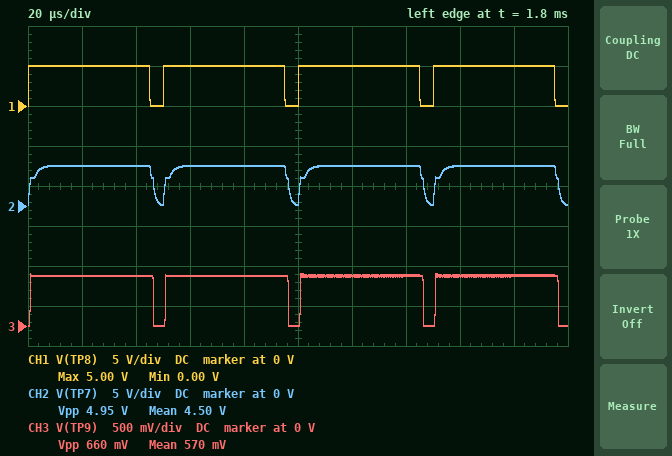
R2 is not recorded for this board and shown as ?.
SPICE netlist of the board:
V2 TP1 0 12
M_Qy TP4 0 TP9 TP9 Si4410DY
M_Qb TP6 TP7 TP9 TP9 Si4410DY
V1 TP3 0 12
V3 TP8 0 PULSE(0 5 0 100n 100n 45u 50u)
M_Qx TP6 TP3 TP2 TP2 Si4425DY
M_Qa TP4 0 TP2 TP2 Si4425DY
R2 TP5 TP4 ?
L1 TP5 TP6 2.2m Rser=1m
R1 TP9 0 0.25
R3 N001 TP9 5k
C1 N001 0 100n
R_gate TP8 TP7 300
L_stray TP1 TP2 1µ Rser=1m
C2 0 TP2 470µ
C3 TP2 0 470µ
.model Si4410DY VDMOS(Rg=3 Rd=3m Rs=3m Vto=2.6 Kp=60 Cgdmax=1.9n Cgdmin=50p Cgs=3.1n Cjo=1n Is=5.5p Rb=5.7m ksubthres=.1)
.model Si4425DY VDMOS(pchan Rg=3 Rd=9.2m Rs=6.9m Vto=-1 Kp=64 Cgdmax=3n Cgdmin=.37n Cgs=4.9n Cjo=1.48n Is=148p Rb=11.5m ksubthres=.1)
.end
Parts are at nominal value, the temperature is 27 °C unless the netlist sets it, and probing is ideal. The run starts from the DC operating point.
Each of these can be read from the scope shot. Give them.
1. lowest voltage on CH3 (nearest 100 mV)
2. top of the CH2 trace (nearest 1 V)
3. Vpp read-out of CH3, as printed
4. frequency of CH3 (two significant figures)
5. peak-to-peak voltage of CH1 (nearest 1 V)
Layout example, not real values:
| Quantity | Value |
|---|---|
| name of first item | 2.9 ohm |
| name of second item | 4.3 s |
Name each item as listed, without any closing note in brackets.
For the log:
| Quantity | Value |
|---|---|
| lowest voltage on CH3 | 0 V |
| top of the CH2 trace | 5 V |
| Vpp read-out of CH3, as printed | 660 mV |
| frequency of CH3 | 20 kHz |
| peak-to-peak voltage of CH1 | 5 V |
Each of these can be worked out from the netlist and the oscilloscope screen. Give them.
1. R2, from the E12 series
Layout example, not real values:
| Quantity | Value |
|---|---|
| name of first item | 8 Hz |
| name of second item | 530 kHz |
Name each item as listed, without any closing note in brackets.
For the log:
| Quantity | Value |
|---|---|
| R2, from the E12 series | 3.9 Ω |
